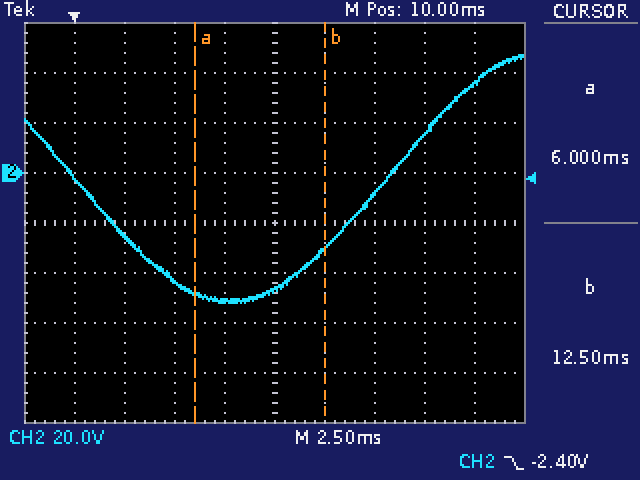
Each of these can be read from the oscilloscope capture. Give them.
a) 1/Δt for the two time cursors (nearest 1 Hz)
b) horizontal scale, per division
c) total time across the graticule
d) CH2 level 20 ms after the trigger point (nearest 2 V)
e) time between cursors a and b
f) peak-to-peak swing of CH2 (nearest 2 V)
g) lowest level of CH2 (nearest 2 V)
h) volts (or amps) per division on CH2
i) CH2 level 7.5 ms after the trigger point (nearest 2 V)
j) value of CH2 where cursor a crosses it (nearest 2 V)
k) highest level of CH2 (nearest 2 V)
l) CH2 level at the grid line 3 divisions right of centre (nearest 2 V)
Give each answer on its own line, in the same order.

154 Hz
2.5 ms
25 ms
36 V
6.50 ms
100 V
-52 V
20 V
-52 V
-48 V
48 V
16 V
